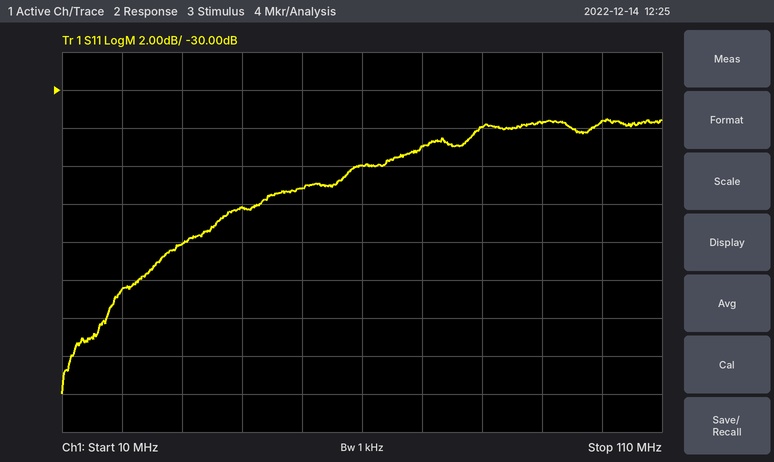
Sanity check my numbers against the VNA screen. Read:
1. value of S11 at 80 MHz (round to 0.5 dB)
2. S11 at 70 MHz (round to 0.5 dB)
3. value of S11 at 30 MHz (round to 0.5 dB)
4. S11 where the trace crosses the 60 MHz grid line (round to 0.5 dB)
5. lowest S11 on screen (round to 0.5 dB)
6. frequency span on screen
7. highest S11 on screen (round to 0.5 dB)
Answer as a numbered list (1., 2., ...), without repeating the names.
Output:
1. -32.0 dB
2. -33.0 dB
3. -38.0 dB
4. -34.0 dB
5. -46.0 dB
6. 100 MHz
7. -31.5 dB
